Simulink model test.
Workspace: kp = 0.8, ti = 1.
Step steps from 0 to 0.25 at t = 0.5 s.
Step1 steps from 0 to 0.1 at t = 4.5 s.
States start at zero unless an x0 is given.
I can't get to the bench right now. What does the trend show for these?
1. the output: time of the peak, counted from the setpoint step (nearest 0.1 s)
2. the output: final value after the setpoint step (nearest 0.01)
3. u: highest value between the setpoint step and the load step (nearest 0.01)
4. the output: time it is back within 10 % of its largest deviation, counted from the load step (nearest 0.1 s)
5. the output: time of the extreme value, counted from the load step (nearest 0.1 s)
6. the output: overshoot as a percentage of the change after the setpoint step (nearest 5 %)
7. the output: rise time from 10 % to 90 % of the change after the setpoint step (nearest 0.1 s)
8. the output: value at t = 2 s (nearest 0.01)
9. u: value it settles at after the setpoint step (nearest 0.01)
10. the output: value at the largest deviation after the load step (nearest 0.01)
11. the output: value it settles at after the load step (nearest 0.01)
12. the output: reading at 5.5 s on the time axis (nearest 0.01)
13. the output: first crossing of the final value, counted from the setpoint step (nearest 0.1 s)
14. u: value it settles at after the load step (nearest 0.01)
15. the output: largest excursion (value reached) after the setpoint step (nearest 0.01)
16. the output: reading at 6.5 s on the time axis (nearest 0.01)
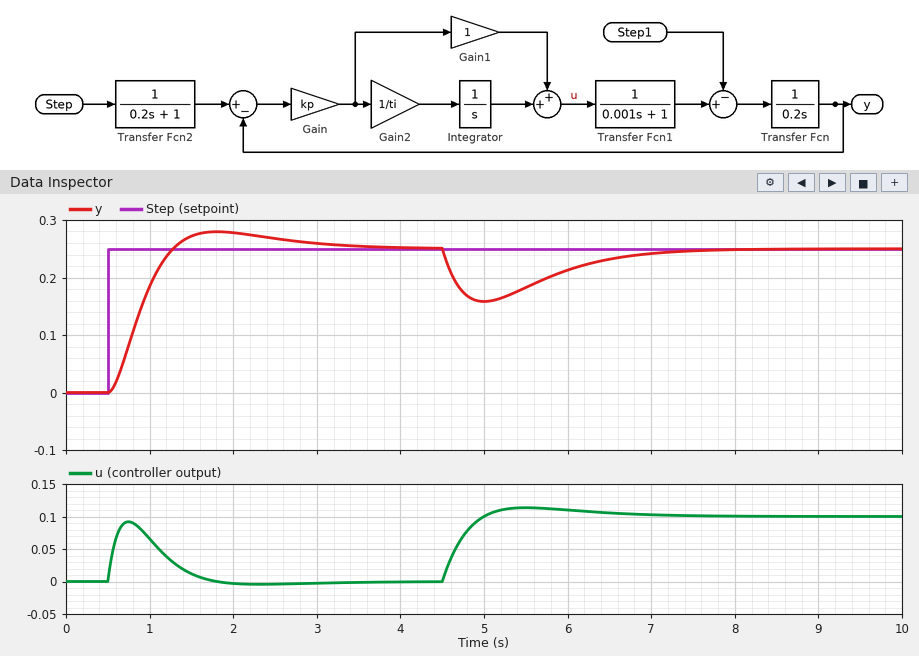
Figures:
1.3 s
0.25
0.09
2.4 s
0.5 s
10 %
0.5 s
0.28
0.00
0.16
0.25
0.18
0.8 s
0.10
0.28
0.23
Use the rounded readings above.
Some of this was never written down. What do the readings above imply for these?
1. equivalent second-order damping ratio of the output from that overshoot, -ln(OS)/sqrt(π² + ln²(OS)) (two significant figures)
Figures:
0.59
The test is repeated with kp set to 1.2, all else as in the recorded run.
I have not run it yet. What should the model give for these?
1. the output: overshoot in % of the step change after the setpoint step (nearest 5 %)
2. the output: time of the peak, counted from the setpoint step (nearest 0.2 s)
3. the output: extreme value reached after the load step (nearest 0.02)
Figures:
10 %
1.2 s
0.18
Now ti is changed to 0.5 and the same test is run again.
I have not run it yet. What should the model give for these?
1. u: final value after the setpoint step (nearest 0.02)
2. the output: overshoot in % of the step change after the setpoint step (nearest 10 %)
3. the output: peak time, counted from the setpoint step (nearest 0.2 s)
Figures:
0.00
20 %
1.0 s
